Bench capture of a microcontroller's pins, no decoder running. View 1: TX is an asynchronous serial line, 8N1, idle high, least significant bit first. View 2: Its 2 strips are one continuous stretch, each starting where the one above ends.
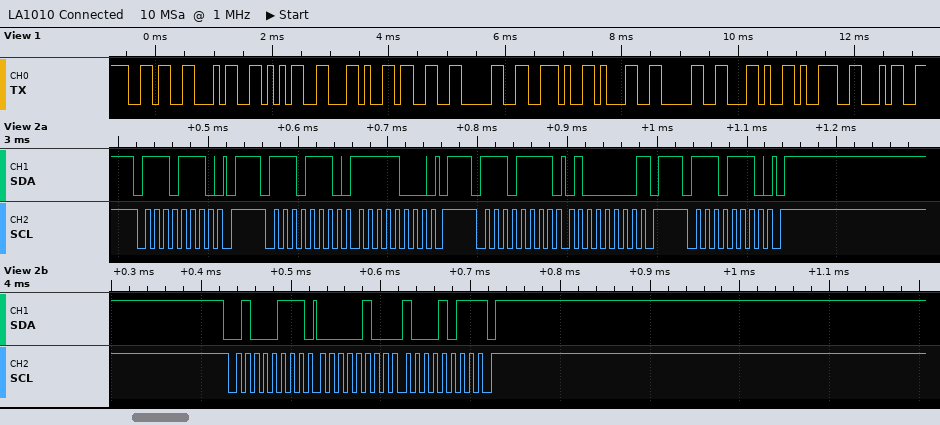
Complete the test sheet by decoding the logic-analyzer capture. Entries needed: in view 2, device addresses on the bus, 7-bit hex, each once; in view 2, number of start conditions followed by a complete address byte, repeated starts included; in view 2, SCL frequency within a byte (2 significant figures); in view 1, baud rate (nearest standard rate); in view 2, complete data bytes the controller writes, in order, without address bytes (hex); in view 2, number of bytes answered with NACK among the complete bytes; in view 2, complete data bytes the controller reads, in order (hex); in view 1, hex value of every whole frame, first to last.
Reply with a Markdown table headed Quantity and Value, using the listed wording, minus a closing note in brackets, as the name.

| Quantity | Value |
|---|---|
| in view 2, device addresses on the bus, 7-bit hex, each once | 0x77 0x23 |
| in view 2, number of start conditions followed by a complete address byte, repeated starts included | 5 |
| in view 2, SCL frequency within a byte | 100 kHz |
| in view 1, baud rate | 9600 baud |
| in view 2, complete data bytes the controller writes, in order, without address bytes | F8 |
| in view 2, number of bytes answered with NACK among the complete bytes | 2 |
| in view 2, complete data bytes the controller reads, in order | 40 04 8B |
| in view 1, hex value of every whole frame, first to last | 36 34 35 2C 33 30 2E 31 30 2C 39 34 |
